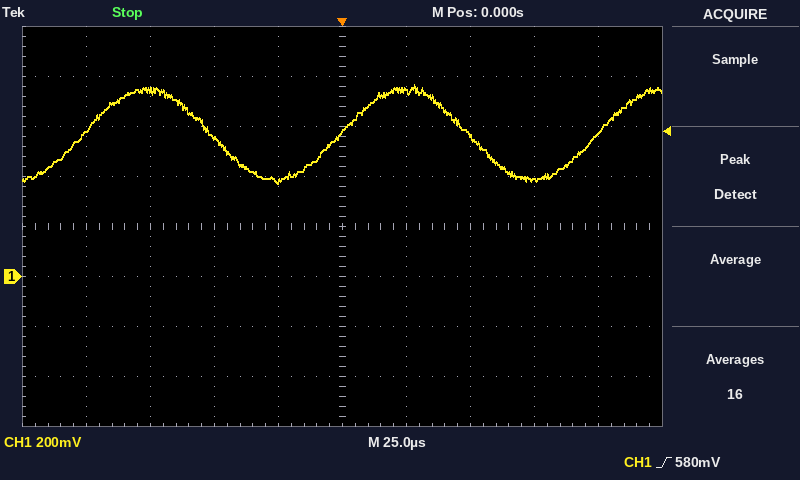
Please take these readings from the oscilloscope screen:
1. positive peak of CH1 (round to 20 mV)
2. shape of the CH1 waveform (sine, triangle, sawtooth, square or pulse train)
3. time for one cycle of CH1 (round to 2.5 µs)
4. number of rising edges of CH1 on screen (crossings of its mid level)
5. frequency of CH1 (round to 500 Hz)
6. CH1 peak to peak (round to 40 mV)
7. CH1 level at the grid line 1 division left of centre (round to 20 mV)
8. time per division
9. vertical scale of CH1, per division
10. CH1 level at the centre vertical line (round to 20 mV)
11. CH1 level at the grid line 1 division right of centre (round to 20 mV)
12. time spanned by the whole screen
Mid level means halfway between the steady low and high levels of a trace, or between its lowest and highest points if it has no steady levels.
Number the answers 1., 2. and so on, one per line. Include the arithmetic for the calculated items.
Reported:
1. 760 mV
2. sine
3. 100.0 µs
4. 3
5. 1 / 100.0 µs ≈ 10.0 kHz
6. 400 mV
7. 380 mV
8. 25 µs
9. 200 mV
10. 580 mV
11. 740 mV
12. 250 µs
